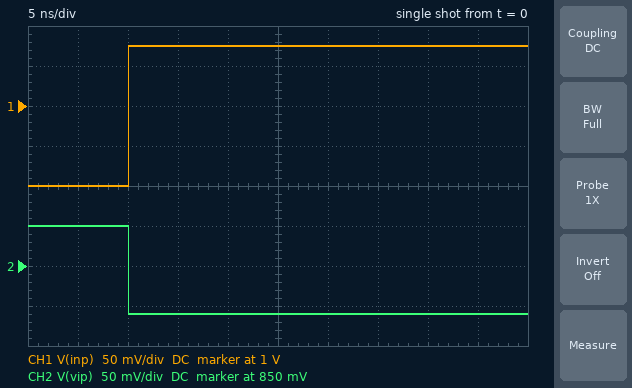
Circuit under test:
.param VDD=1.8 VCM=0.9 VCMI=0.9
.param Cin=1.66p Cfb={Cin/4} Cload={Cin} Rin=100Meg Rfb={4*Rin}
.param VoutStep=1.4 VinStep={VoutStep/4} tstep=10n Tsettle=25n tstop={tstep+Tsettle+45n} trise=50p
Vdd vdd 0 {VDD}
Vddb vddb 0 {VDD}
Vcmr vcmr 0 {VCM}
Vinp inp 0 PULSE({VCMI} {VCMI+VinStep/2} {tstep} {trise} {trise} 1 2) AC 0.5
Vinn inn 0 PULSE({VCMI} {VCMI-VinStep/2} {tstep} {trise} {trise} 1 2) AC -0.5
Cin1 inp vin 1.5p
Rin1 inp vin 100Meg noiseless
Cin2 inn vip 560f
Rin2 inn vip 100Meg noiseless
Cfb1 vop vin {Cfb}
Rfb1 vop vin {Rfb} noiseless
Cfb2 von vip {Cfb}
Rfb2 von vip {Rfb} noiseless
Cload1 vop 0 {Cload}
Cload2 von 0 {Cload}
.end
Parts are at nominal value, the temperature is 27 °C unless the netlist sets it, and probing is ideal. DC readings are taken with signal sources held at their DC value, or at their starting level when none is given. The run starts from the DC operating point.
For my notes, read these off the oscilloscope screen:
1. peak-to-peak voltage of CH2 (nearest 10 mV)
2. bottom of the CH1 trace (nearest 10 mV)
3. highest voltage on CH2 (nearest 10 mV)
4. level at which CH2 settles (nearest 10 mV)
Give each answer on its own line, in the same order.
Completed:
110 mV
900 mV
900 mV
790 mV
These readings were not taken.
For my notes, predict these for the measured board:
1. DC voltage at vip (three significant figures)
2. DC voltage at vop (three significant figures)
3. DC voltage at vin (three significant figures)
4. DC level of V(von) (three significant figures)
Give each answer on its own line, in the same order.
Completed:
900 mV
900 mV
900 mV
900 mV
